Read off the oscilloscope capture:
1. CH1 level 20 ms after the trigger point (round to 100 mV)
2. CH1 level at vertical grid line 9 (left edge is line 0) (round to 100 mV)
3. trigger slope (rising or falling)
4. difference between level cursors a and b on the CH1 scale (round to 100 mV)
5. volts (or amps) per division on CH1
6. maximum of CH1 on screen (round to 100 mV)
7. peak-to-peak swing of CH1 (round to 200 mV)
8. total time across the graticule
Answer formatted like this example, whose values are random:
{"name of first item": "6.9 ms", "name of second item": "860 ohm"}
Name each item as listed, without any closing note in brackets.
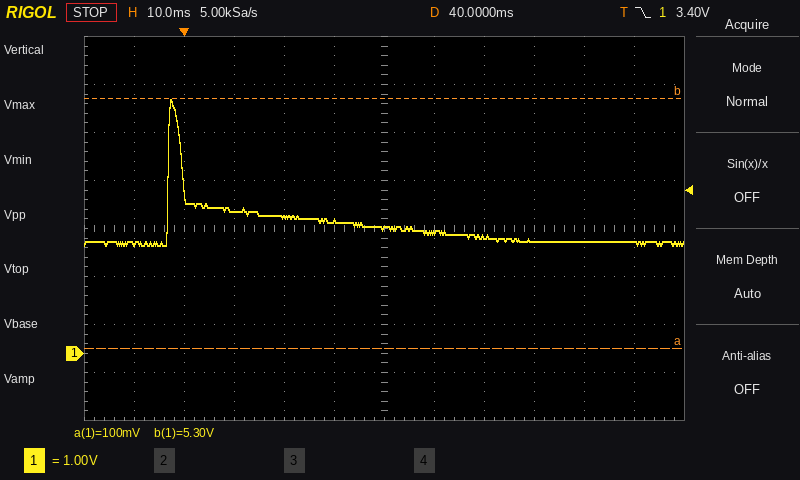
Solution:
{"CH1 level 20 ms after the trigger point": "2.8 V", "CH1 level at vertical grid line 9 (left edge is line 0)": "2.3 V", "trigger slope": "falling", "difference between level cursors a and b on the CH1 scale": "5.2 V", "volts (or amps) per division on CH1": "1 V", "maximum of CH1 on screen": "5.3 V", "peak-to-peak swing of CH1": "3.0 V", "total time across the graticule": "120 ms"}
